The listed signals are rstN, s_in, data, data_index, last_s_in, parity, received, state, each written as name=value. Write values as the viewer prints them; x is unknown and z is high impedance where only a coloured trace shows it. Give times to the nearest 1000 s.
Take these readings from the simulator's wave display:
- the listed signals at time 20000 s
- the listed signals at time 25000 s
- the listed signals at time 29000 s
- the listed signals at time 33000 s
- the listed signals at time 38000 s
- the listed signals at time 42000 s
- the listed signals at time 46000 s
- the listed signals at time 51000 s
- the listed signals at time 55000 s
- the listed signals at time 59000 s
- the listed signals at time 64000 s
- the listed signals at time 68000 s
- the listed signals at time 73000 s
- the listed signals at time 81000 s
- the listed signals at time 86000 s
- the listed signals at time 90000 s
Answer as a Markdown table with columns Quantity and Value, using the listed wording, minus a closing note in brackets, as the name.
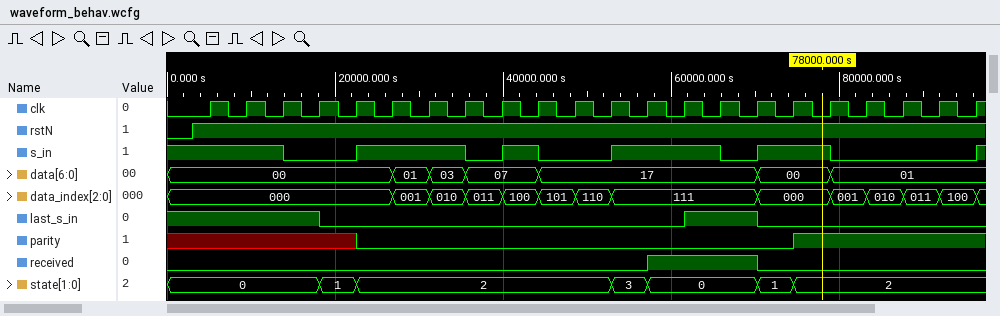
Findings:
| Quantity | Value |
|---|---|
| the listed signals at time 20000 s | rstN=1, s_in=0, data=00, data_index=000, last_s_in=0, parity=x, received=0, state=1 |
| the listed signals at time 25000 s | rstN=1, s_in=1, data=00, data_index=000, last_s_in=0, parity=0, received=0, state=2 |
| the listed signals at time 29000 s | rstN=1, s_in=1, data=01, data_index=001, last_s_in=0, parity=0, received=0, state=2 |
| the listed signals at time 33000 s | rstN=1, s_in=1, data=03, data_index=010, last_s_in=0, parity=0, received=0, state=2 |
| the listed signals at time 38000 s | rstN=1, s_in=0, data=07, data_index=011, last_s_in=0, parity=0, received=0, state=2 |
| the listed signals at time 42000 s | rstN=1, s_in=1, data=07, data_index=100, last_s_in=0, parity=0, received=0, state=2 |
| the listed signals at time 46000 s | rstN=1, s_in=0, data=17, data_index=101, last_s_in=0, parity=0, received=0, state=2 |
| the listed signals at time 51000 s | rstN=1, s_in=0, data=17, data_index=110, last_s_in=0, parity=0, received=0, state=2 |
| the listed signals at time 55000 s | rstN=1, s_in=1, data=17, data_index=111, last_s_in=0, parity=0, received=0, state=3 |
| the listed signals at time 59000 s | rstN=1, s_in=1, data=17, data_index=111, last_s_in=0, parity=0, received=1, state=0 |
| the listed signals at time 64000 s | rstN=1, s_in=1, data=17, data_index=111, last_s_in=1, parity=0, received=1, state=0 |
| the listed signals at time 68000 s | rstN=1, s_in=0, data=17, data_index=111, last_s_in=1, parity=0, received=1, state=0 |
| the listed signals at time 73000 s | rstN=1, s_in=1, data=00, data_index=000, last_s_in=0, parity=0, received=0, state=1 |
| the listed signals at time 81000 s | rstN=1, s_in=0, data=01, data_index=001, last_s_in=0, parity=1, received=0, state=2 |
| the listed signals at time 86000 s | rstN=1, s_in=0, data=01, data_index=010, last_s_in=0, parity=1, received=0, state=2 |
| the listed signals at time 90000 s | rstN=1, s_in=0, data=01, data_index=011, last_s_in=0, parity=1, received=0, state=2 |
